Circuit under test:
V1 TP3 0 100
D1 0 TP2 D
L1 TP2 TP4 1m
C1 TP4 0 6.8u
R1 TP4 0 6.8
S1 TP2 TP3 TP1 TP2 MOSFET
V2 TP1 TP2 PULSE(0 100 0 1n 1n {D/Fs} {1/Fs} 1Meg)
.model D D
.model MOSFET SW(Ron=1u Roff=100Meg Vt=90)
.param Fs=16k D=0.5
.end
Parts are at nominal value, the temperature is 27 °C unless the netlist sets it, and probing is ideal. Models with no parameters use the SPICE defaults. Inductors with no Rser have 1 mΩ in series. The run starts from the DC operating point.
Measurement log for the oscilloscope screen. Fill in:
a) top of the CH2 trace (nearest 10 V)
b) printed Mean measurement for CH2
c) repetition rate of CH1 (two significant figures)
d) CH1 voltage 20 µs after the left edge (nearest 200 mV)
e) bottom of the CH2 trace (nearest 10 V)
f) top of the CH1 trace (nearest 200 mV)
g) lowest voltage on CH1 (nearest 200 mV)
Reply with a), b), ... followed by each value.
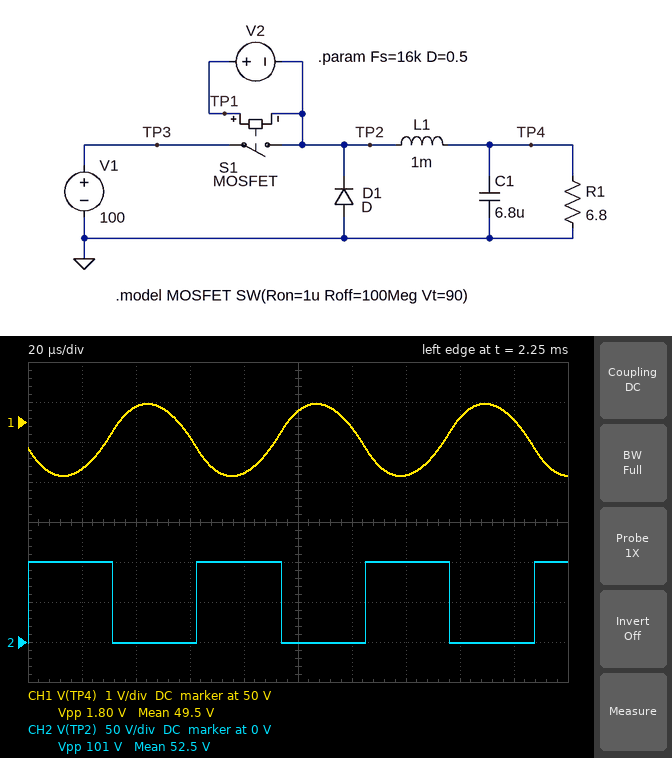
a) 100 V
b) 52.5 V
c) 16 kHz
d) 48.8 V
e) 0 V
f) 50.4 V
g) 48.6 V
